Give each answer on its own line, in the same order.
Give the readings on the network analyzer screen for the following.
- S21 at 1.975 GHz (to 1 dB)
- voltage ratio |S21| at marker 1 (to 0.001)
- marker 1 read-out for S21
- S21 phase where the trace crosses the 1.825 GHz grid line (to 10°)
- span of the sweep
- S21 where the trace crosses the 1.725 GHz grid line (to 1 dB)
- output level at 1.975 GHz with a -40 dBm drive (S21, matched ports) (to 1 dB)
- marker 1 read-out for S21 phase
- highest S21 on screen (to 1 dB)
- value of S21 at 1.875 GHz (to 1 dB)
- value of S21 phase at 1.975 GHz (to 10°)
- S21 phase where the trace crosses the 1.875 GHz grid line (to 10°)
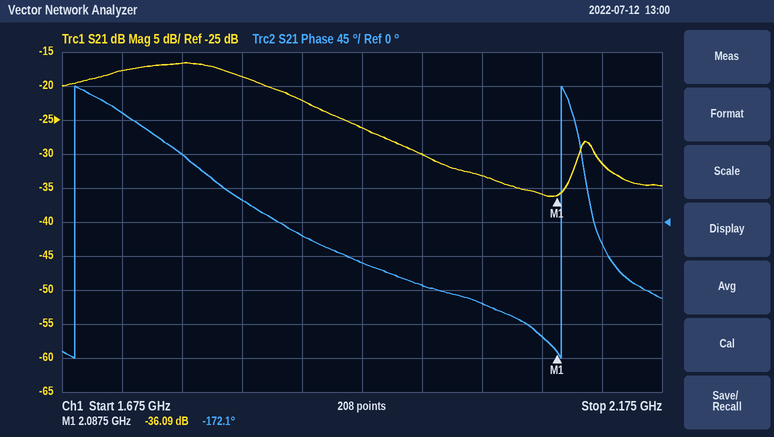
-30 dB
0.016
-36.09 dB
30°
500 MHz
-18 dB
-70 dBm
-172.1°
-17 dB
-22 dB
-80°
-20°
